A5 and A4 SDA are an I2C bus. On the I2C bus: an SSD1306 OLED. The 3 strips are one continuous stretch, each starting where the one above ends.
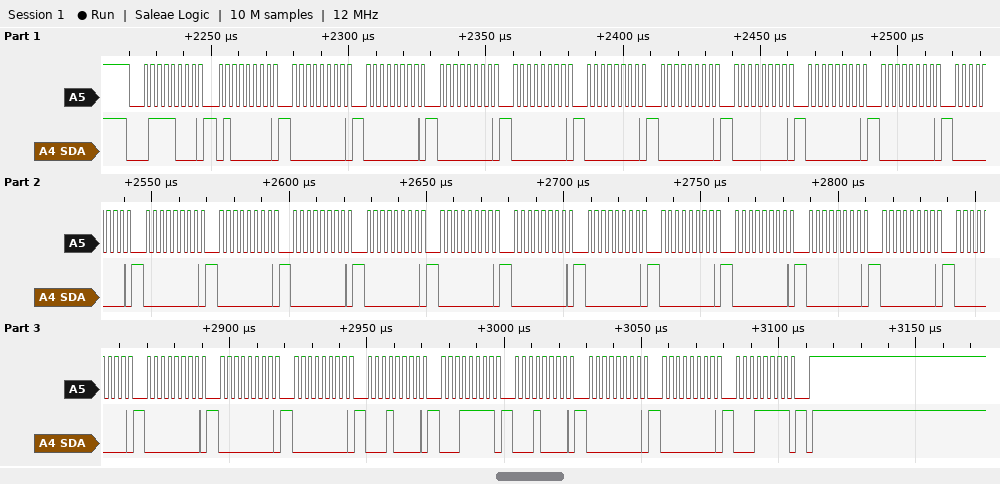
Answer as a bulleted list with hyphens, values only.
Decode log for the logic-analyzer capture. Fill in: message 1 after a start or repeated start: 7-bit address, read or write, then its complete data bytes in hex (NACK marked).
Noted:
- 0x3C write: 40 00 00 00 00 00 00 00 00 00 00 00 00 00 00 00 00 00 00 00 00 00 00 00 00 00 10 1F 10 00 00 1F
